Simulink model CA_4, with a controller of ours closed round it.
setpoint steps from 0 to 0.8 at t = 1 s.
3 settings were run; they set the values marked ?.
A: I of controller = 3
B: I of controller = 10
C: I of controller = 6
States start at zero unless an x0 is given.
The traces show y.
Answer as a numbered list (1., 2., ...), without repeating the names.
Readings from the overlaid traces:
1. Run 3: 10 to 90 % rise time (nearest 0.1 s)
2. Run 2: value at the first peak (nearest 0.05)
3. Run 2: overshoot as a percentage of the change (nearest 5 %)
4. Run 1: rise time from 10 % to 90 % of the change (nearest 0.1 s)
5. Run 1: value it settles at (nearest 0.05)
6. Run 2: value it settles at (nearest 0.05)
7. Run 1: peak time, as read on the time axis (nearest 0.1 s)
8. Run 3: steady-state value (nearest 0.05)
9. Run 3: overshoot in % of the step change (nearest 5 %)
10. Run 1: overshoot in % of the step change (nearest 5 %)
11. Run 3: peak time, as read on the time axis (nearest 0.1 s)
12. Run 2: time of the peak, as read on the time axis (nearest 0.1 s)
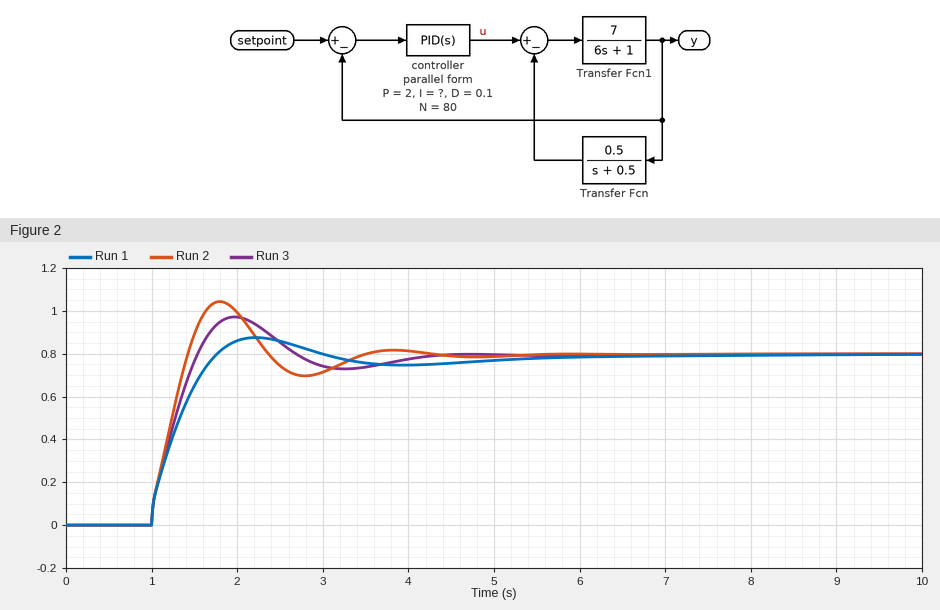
1. 0.4 s
2. 1.05
3. 30 %
4. 0.6 s
5. 0.80
6. 0.80
7. 2.2 s
8. 0.80
9. 20 %
10. 10 %
11. 2.0 s
12. 1.8 s
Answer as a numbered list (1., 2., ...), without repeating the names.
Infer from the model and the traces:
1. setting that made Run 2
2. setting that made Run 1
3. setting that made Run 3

1. B
2. A
3. C
